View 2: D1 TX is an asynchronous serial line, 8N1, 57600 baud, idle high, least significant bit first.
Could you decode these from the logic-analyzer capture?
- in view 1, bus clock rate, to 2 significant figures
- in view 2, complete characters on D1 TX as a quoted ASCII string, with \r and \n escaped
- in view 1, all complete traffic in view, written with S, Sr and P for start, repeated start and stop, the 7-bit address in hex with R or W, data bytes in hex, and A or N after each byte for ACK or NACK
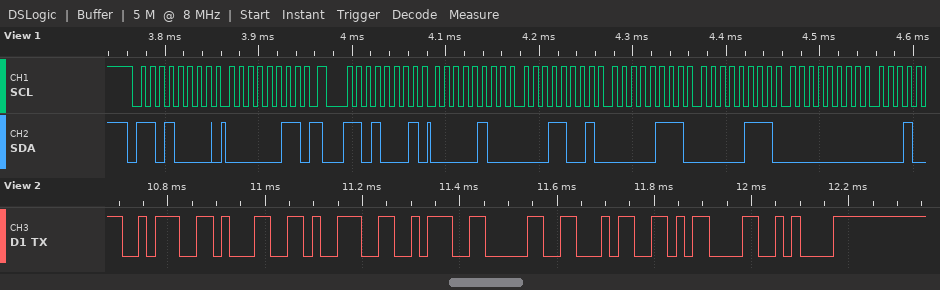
100 kHz
":19:04\r\n"
S 68W A 03 A Sr 68R A 04 A 19 A 07 A 07 A 00 A
